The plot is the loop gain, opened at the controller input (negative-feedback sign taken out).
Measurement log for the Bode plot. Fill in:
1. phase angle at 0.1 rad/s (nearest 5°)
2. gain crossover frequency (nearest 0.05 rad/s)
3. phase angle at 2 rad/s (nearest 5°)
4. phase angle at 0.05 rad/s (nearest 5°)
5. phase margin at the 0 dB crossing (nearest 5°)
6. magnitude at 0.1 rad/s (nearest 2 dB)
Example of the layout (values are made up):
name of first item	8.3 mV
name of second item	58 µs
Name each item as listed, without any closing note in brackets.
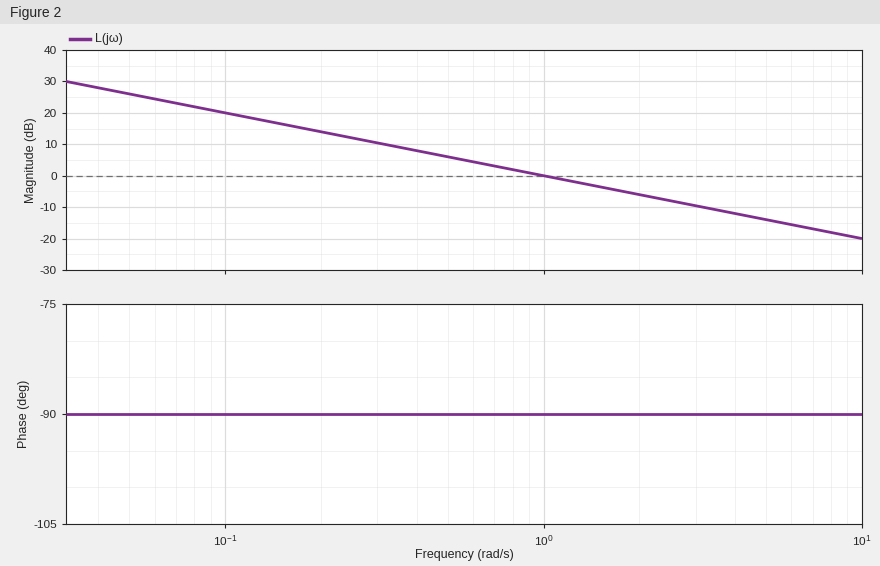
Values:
phase angle at 0.1 rad/s	-90°
gain crossover frequency	1.00 rad/s
phase angle at 2 rad/s	-90°
phase angle at 0.05 rad/s	-90°
phase margin at the 0 dB crossing	90°
magnitude at 0.1 rad/s	20 dB
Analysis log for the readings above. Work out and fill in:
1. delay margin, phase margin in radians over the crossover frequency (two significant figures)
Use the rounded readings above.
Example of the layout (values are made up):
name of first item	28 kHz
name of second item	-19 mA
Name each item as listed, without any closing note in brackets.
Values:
delay margin, phase margin in radians over the crossover frequency	1.6 s
